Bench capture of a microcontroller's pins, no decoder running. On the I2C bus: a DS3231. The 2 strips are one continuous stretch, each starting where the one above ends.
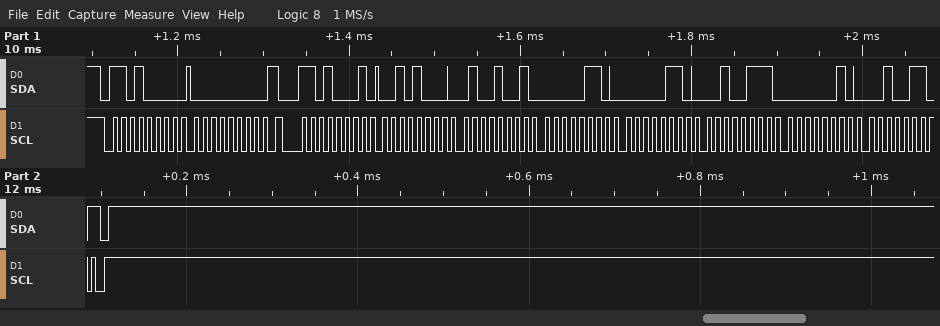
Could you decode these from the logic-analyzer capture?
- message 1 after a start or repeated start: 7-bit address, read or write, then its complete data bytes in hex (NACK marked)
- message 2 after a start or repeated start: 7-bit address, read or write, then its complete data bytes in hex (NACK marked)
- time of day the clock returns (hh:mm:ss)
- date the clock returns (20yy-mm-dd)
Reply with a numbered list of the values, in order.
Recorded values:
1. 0x68 write: 00
2. 0x68 read: 28 49 06 06 27 02 26 NACK
3. 06:49:28
4. 2026-02-27
